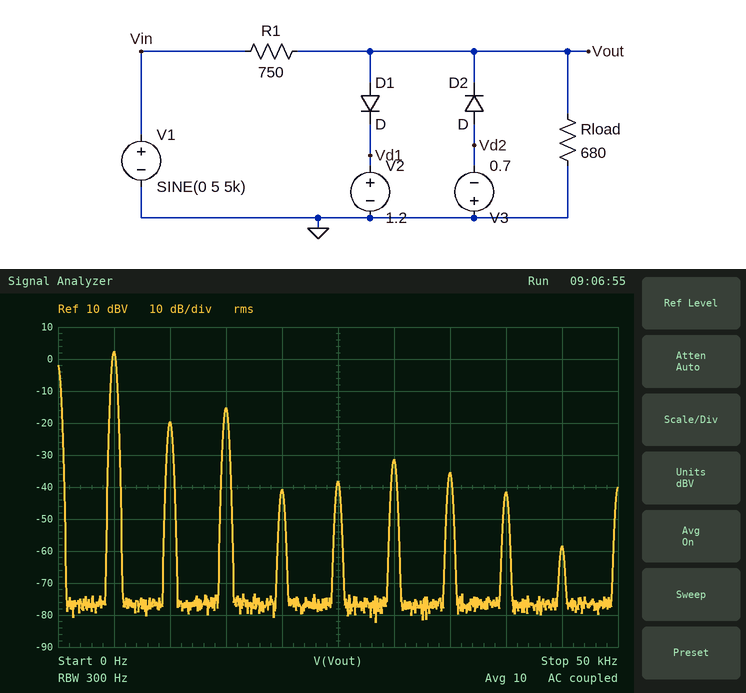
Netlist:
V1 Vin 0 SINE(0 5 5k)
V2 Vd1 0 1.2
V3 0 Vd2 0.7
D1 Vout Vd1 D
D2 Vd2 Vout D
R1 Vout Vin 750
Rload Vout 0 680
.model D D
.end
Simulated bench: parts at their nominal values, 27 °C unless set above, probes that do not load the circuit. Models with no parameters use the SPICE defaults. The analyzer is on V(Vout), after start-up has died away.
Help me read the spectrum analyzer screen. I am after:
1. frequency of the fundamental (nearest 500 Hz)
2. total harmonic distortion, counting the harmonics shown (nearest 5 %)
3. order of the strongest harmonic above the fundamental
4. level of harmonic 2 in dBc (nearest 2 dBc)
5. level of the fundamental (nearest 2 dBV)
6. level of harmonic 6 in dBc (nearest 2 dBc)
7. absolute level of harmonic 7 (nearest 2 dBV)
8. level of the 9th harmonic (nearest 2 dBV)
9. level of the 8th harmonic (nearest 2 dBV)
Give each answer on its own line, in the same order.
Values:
5.0 kHz
15 %
3
-22 dBc
2 dBV
-34 dBc
-36 dBV
-58 dBV
-42 dBV
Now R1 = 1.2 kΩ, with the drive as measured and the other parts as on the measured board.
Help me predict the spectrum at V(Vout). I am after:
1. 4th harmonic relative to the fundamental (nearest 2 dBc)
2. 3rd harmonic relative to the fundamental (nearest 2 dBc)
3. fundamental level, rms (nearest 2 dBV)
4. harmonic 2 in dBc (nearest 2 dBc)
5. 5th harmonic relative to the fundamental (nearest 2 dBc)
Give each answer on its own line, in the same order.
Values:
-32 dBc
-26 dBc
2 dBV
-24 dBc
-38 dBc
